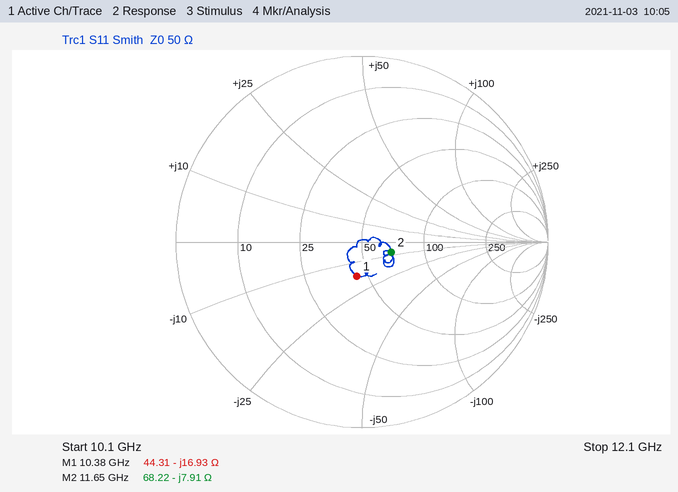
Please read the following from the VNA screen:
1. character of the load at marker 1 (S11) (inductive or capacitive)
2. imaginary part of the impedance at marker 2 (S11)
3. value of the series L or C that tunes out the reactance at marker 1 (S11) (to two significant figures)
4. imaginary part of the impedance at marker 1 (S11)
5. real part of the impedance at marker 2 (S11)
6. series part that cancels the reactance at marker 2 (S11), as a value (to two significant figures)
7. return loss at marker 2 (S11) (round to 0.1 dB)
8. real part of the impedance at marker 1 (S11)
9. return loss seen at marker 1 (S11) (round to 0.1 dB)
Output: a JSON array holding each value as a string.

["capacitive", "-7.91 Ω", "260 pH", "-16.93 Ω", "68.22 Ω", "110 pH", "15.5 dB", "44.31 Ω", "14.6 dB"]
